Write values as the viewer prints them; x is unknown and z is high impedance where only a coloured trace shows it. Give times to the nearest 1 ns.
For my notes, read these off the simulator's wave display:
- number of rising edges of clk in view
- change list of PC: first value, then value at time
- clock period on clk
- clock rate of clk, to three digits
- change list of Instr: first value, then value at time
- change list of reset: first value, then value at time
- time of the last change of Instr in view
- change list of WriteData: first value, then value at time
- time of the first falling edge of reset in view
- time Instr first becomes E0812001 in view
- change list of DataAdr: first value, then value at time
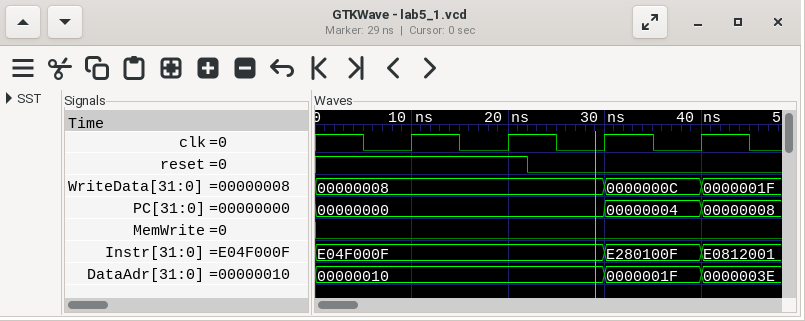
4
00000000, 00000004 at 30 ns, 00000008 at 40 ns
10 ns
100 MHz
E04F000F, E280100F at 30 ns, E0812001 at 40 ns
1, 0 at 22 ns
40 ns
00000008, 0000000C at 30 ns, 0000001F at 40 ns
22 ns
40 ns
00000010, 0000001F at 30 ns, 0000003E at 40 ns
